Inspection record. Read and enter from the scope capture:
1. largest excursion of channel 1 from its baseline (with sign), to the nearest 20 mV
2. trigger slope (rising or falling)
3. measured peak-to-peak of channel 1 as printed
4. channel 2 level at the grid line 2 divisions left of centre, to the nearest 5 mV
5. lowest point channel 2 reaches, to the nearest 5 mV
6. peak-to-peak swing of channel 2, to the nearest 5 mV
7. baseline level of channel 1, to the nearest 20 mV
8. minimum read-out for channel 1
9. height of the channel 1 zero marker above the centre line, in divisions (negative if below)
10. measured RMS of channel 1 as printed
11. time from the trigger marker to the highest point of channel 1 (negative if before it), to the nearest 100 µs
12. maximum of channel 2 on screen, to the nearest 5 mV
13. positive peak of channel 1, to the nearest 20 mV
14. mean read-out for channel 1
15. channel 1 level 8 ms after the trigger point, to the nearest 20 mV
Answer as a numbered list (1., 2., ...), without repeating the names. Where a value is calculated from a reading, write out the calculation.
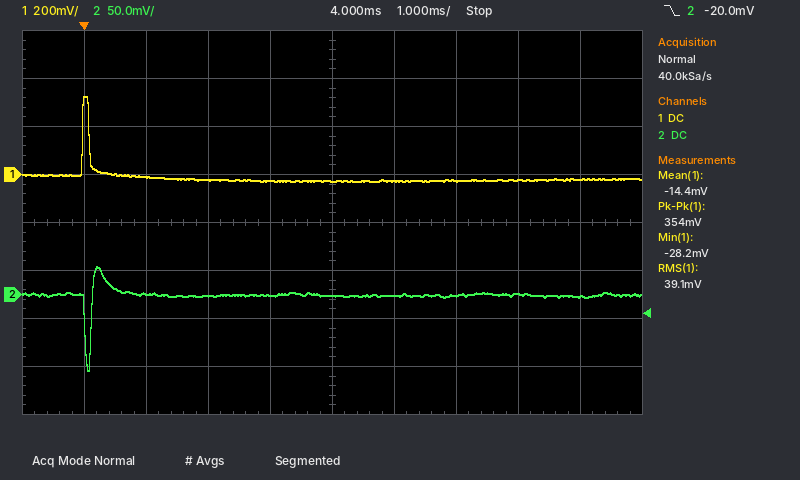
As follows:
1. 320 mV − (-20 mV) = +340 mV
2. falling
3. 354 mV
4. 0 mV
5. -80 mV
6. 30 mV − (-80 mV) = 110 mV
7. -20 mV
8. -28.2 mV
9. +1.0 div
10. 39.1 mV
11. 0.0 ms
12. 30 mV
13. 320 mV
14. -14.4 mV
15. -20 mV
